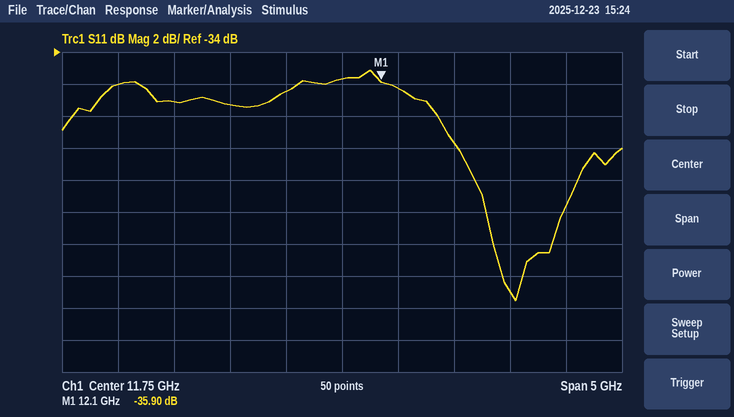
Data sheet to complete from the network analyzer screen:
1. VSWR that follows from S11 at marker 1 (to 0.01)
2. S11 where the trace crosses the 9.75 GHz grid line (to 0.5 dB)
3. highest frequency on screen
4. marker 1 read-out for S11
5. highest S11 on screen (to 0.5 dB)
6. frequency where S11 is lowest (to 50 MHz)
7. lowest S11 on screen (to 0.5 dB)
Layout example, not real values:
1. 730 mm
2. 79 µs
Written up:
1. 1.03
2. -36.0 dB
3. 14.25 GHz
4. -35.90 dB
5. -35.0 dB
6. 13.30 GHz
7. -49.5 dB
